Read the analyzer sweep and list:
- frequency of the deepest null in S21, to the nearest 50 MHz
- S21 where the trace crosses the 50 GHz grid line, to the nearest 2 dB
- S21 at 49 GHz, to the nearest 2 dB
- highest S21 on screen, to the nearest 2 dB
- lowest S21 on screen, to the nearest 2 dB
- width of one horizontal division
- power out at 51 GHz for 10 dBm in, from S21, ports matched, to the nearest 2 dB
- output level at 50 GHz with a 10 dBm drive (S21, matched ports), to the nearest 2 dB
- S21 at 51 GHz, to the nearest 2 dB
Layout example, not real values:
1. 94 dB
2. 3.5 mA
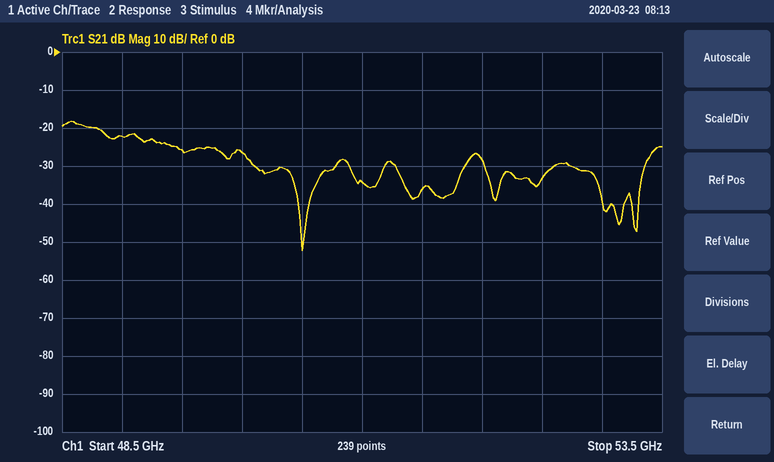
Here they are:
1. 50.50 GHz
2. -26 dB
3. -22 dB
4. -18 dB
5. -52 dB
6. 500 MHz
7. -24 dBm
8. -16 dBm
9. -34 dB
